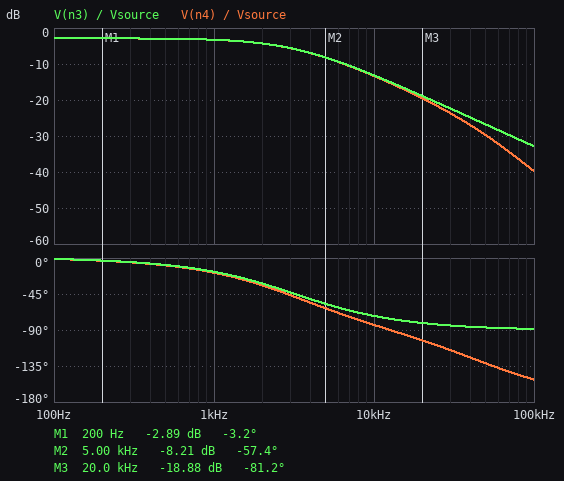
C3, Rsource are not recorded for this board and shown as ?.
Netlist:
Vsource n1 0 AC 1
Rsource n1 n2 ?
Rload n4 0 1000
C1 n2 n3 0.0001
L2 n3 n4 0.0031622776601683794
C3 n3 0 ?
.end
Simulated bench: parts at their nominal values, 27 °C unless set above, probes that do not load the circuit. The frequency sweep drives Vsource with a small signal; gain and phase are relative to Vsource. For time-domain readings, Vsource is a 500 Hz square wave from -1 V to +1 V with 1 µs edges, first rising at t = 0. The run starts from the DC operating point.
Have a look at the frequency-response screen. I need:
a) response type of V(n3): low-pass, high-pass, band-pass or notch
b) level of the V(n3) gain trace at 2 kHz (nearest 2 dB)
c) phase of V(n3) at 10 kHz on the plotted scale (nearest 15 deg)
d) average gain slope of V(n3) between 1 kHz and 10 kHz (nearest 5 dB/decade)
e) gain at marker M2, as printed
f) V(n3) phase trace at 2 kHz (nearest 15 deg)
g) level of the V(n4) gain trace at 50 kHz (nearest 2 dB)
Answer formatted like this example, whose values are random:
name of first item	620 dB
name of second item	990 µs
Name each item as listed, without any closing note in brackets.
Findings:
response type of V(n3): low-pass, high-pass, band-pass or notch	low-pass
level of the V(n3) gain trace at 2 kHz	-4 dB
phase of V(n3) at 10 kHz on the plotted scale	-75 deg
average gain slope of V(n3) between 1 kHz and 10 kHz	-10 dB/decade
gain at marker M2, as printed	-8.21 dB
V(n3) phase trace at 2 kHz	-30 deg
level of the V(n4) gain trace at 50 kHz	-30 dB
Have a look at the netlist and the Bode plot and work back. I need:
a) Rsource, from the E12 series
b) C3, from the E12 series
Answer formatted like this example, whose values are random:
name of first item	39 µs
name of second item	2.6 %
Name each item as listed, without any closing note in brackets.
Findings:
Rsource, from the E12 series	390 Ω
C3, from the E12 series	180 nF
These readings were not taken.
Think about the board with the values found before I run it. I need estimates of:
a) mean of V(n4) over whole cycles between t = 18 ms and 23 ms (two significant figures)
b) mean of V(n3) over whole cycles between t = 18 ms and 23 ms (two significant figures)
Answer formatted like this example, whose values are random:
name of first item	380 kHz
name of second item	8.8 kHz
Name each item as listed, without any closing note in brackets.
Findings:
mean of V(n4) over whole cycles between t = 18 ms and 23 ms	620 mV
mean of V(n3) over whole cycles between t = 18 ms and 23 ms	620 mV
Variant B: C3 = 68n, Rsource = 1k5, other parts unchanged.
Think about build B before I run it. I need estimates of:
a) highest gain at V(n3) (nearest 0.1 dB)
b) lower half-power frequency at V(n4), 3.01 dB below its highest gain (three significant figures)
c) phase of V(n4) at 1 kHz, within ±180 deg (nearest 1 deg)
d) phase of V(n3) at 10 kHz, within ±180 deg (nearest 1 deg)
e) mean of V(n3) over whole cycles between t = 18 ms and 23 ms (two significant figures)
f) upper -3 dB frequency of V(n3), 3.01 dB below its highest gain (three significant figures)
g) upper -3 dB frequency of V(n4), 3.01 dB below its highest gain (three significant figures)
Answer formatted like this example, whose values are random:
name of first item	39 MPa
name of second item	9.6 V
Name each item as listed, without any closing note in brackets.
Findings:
highest gain at V(n3)	-8.0 dB
lower half-power frequency at V(n4), 3.01 dB below its highest gain	636 mHz
phase of V(n4) at 1 kHz, within ±180 deg	-15 deg
phase of V(n3) at 10 kHz, within ±180 deg	-68 deg
mean of V(n3) over whole cycles between t = 18 ms and 23 ms	370 mV
upper -3 dB frequency of V(n3), 3.01 dB below its highest gain	4.11 kHz
upper -3 dB frequency of V(n4), 3.01 dB below its highest gain	4.08 kHz
